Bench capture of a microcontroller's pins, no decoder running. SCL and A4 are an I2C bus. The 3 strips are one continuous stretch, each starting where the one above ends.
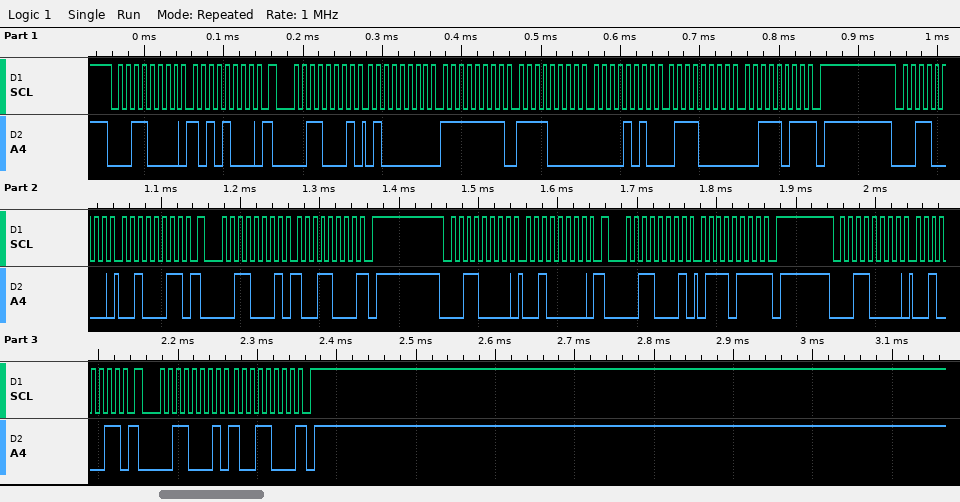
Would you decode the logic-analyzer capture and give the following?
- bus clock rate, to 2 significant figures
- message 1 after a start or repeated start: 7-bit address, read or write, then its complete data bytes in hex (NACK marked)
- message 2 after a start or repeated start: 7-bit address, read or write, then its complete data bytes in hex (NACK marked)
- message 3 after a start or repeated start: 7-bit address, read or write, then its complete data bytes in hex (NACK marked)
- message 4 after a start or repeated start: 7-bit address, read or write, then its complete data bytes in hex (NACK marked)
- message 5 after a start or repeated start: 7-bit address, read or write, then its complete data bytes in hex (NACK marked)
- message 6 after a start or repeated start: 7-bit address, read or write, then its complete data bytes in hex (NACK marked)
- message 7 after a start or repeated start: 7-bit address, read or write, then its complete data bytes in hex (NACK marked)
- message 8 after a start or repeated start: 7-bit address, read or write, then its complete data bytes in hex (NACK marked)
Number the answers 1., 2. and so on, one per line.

1. 100 kHz
2. 0x18 write: A8
3. 0x18 read: 40 FF F0 0A 70 3B NACK
4. 0x18 write: 23
5. 0x18 read: 98 NACK
6. 0x18 write: 20
7. 0x18 read: 77 NACK
8. 0x18 write: 23
9. 0x18 read: 98 NACK
